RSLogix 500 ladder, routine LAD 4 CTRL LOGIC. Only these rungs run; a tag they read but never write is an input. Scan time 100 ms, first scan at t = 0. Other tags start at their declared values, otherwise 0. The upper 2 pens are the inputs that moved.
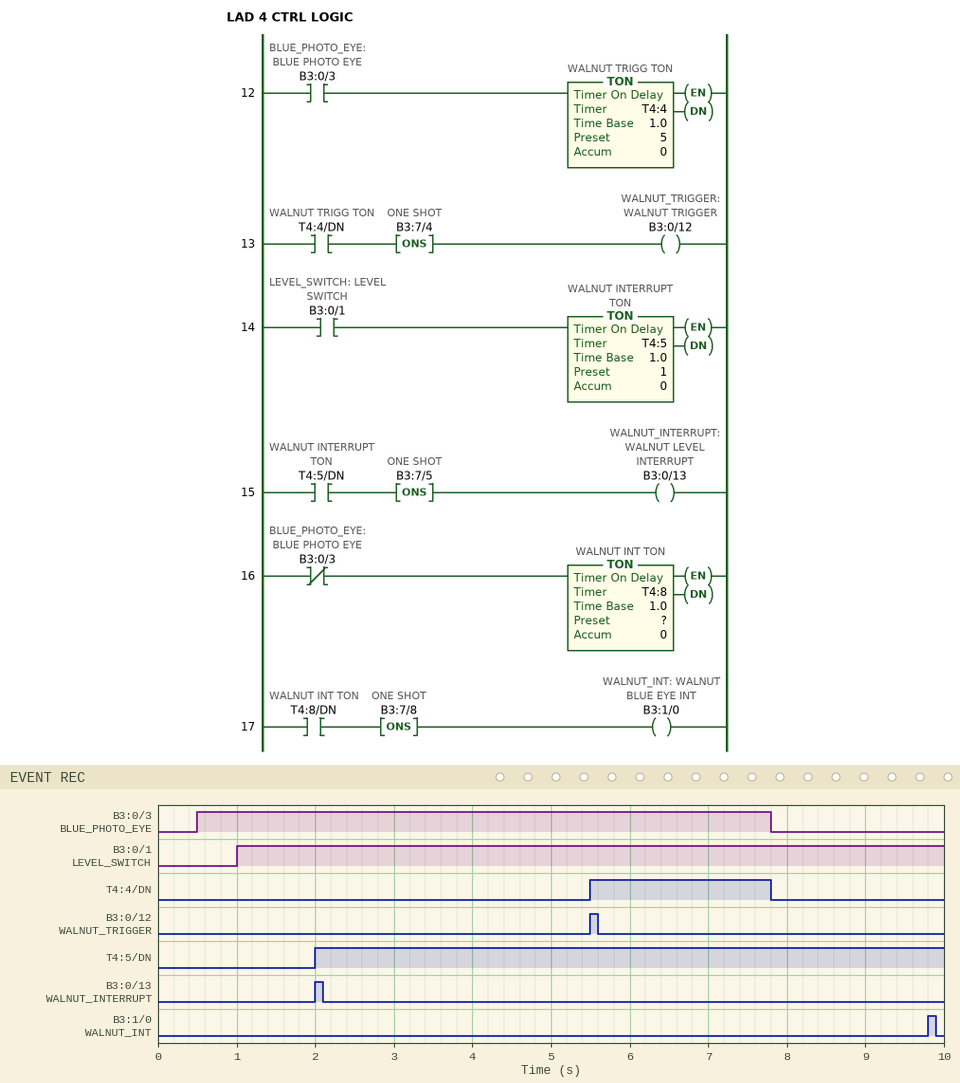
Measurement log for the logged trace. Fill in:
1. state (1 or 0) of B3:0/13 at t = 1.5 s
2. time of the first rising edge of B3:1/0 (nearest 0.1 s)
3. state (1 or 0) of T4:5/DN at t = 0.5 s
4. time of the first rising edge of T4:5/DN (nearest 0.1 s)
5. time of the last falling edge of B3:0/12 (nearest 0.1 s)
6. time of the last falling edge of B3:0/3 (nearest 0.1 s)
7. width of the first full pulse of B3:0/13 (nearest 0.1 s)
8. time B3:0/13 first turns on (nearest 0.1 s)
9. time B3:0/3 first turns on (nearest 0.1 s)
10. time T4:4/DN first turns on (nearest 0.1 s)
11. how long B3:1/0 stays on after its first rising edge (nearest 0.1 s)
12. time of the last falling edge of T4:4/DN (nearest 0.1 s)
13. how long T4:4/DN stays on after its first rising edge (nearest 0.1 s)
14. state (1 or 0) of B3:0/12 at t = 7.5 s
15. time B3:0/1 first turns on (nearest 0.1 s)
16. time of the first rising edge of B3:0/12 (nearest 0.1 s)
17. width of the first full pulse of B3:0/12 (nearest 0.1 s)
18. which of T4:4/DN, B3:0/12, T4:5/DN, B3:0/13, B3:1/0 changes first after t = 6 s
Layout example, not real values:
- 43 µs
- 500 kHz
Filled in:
- 0
- 9.8 s
- 0
- 2.0 s
- 5.6 s
- 7.8 s
- 0.1 s
- 2.0 s
- 0.5 s
- 5.5 s
- 0.1 s
- 7.8 s
- 2.3 s
- 0
- 1.0 s
- 5.5 s
- 0.1 s
- T4:4/DN
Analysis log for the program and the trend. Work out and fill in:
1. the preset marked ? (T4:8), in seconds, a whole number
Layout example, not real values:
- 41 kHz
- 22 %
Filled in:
- 2 s
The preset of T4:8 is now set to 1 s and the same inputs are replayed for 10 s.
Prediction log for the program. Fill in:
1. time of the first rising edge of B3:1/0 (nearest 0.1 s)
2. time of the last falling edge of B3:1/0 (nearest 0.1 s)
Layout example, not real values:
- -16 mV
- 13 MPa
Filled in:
- 8.8 s
- 8.9 s
